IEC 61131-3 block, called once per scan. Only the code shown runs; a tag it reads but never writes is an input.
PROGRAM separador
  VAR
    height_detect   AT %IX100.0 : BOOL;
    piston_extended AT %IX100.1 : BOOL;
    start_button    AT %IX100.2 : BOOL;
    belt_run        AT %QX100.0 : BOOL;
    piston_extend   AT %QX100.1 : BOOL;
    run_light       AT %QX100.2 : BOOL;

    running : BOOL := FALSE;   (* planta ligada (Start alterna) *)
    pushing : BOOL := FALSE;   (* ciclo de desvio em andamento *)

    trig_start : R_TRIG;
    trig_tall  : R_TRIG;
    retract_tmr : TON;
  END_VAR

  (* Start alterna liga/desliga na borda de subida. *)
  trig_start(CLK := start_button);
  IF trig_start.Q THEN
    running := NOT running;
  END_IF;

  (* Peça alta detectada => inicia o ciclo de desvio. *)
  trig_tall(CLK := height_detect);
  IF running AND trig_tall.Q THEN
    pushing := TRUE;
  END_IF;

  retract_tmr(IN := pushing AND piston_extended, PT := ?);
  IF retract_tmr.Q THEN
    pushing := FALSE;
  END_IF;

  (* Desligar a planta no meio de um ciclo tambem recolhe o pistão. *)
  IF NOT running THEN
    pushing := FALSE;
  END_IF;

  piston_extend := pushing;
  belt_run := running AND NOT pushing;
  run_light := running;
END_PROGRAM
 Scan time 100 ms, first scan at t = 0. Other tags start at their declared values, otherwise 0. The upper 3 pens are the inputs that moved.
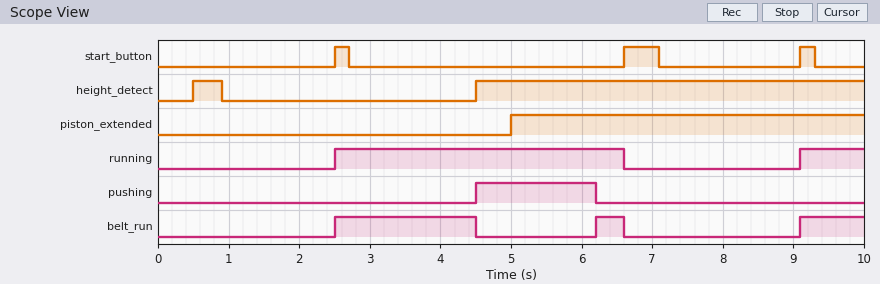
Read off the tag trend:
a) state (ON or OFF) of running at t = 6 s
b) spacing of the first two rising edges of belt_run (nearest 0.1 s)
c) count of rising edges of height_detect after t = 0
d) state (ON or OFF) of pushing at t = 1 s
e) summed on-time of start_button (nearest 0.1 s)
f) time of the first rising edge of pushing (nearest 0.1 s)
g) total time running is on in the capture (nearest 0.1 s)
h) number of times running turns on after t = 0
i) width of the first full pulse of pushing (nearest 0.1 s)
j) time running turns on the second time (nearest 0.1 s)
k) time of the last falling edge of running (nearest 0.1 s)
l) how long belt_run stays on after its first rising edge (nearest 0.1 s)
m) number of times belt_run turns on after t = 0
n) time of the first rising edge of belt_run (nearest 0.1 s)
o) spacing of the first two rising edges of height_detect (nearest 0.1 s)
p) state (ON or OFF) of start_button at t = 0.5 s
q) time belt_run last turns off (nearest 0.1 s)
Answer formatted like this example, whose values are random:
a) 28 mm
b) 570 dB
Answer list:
a) ON
b) 3.7 s
c) 2
d) OFF
e) 0.9 s
f) 4.5 s
g) 5.0 s
h) 2
i) 1.7 s
j) 9.1 s
k) 6.6 s
l) 2.0 s
m) 3
n) 2.5 s
o) 4.0 s
p) OFF
q) 6.6 s
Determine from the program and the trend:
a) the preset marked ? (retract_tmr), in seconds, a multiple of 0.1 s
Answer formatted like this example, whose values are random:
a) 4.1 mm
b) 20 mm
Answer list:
a) 1.2 s
